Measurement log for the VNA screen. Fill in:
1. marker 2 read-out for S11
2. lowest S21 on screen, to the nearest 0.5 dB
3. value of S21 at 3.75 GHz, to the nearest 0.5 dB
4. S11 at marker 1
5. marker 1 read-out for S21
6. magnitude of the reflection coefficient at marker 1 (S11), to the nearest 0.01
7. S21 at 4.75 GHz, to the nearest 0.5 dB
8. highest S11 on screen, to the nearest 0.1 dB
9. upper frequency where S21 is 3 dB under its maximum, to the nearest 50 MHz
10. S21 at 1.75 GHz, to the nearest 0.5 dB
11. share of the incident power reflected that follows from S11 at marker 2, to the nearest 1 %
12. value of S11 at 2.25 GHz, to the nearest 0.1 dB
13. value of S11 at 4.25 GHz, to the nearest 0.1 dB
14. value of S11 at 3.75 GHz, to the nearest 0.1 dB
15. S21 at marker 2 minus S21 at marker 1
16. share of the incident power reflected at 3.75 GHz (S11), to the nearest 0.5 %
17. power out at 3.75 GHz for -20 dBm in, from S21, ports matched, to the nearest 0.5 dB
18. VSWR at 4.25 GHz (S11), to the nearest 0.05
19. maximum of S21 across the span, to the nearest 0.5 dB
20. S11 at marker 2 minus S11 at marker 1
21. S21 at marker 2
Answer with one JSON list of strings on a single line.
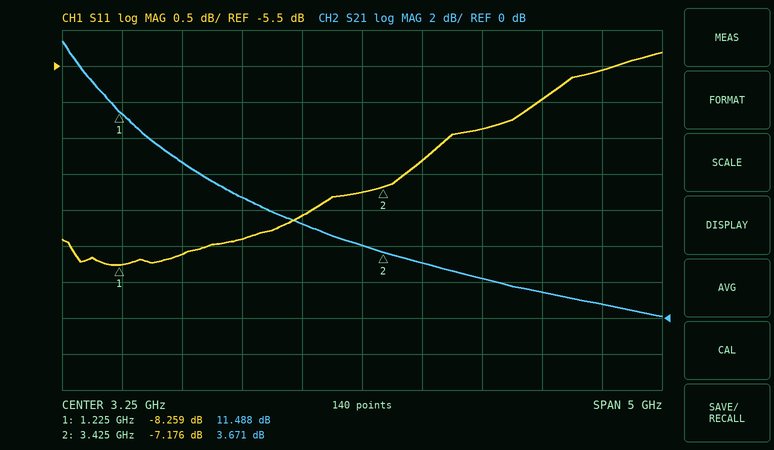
["-7.176 dB", "0.0 dB", "3.0 dB", "-8.259 dB", "11.488 dB", "0.39", "1.5 dB", "-5.3 dB", "1.10 GHz", "8.5 dB", "19 %", "-7.9 dB", "-6.4 dB", "-6.8 dB", "-7.817 dB", "21.0 %", "-17.0 dBm", "2.85", "15.5 dB", "1.083 dB", "3.671 dB"]
